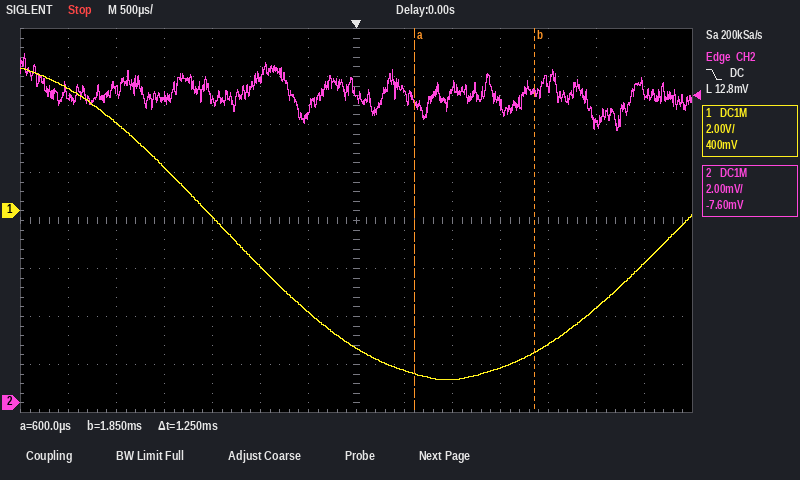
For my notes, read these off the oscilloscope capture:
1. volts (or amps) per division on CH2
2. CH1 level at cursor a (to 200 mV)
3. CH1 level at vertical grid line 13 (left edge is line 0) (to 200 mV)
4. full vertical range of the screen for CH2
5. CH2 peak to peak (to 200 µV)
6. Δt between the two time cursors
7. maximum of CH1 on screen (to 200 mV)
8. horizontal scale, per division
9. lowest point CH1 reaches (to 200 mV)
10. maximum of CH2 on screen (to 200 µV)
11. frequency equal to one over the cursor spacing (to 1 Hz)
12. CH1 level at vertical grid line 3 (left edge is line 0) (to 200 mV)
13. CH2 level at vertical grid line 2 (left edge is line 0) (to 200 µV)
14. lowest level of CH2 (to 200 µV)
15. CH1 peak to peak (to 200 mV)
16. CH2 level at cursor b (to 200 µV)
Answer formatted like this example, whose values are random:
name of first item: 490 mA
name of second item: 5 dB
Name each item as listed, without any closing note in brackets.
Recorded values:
volts (or amps) per division on CH2: 2 mV
CH1 level at cursor a: -6.8 V
CH1 level at vertical grid line 13 (left edge is line 0): -2.2 V
full vertical range of the screen for CH2: 16 mV
CH2 peak to peak: 3.2 mV
Δt between the two time cursors: 1.25 ms
maximum of CH1 on screen: 6.0 V
horizontal scale, per division: 500 µs
lowest point CH1 reaches: -7.0 V
maximum of CH2 on screen: 14.6 mV
frequency equal to one over the cursor spacing: 800 Hz
CH1 level at vertical grid line 3 (left edge is line 0): 1.8 V
CH2 level at vertical grid line 2 (left edge is line 0): 13.0 mV
lowest level of CH2: 11.4 mV
CH1 peak to peak: 13.0 V
CH2 level at cursor b: 13.0 mV
